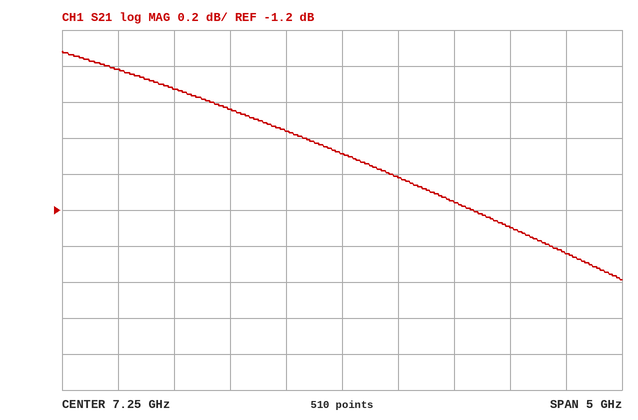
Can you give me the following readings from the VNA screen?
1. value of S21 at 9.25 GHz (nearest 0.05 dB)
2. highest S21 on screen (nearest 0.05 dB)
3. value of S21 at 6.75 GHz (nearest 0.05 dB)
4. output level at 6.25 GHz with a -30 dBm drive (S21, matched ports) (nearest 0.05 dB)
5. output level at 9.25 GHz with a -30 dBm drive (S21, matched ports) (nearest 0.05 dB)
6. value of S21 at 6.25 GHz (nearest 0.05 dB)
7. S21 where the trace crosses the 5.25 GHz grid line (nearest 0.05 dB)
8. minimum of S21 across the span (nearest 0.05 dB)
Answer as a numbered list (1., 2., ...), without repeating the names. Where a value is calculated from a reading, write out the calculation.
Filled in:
1. -1.45 dB
2. -0.30 dB
3. -0.75 dB
4. -30 dBm + (-0.65 dB) = -30.65 dBm
5. -30 dBm + (-1.45 dB) = -31.45 dBm
6. -0.65 dB
7. -0.40 dB
8. -1.60 dB
